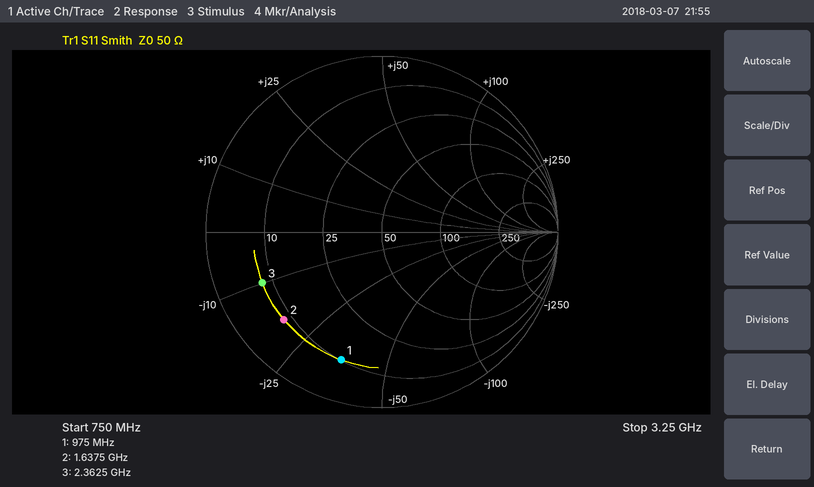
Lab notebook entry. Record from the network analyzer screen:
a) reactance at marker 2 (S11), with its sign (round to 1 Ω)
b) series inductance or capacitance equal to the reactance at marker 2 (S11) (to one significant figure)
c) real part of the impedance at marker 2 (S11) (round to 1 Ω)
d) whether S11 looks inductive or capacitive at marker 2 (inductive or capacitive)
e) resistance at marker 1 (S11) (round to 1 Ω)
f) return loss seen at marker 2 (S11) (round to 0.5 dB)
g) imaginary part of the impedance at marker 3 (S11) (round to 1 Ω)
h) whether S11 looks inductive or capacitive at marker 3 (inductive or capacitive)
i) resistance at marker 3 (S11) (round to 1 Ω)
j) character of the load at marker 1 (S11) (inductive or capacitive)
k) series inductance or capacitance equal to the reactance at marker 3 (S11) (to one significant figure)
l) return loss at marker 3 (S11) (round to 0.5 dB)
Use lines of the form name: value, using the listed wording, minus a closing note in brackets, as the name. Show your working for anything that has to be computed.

reactance at marker 2 (S11), with its sign: -19 Ω
series inductance or capacitance equal to the reactance at marker 2 (S11): C = 1/(2π × 1.6375 GHz × 19 Ω) ≈ 5 pF
real part of the impedance at marker 2 (S11): 8 Ω
whether S11 looks inductive or capacitive at marker 2: capacitive
resistance at marker 1 (S11): 10 Ω
return loss seen at marker 2 (S11): 2.5 dB
imaginary part of the impedance at marker 3 (S11): -10 Ω
whether S11 looks inductive or capacitive at marker 3: capacitive
resistance at marker 3 (S11): 8 Ω
character of the load at marker 1 (S11): capacitive
series inductance or capacitance equal to the reactance at marker 3 (S11): C = 1/(2π × 2.3625 GHz × 10 Ω) ≈ 7 pF
return loss at marker 3 (S11): 2.5 dB
